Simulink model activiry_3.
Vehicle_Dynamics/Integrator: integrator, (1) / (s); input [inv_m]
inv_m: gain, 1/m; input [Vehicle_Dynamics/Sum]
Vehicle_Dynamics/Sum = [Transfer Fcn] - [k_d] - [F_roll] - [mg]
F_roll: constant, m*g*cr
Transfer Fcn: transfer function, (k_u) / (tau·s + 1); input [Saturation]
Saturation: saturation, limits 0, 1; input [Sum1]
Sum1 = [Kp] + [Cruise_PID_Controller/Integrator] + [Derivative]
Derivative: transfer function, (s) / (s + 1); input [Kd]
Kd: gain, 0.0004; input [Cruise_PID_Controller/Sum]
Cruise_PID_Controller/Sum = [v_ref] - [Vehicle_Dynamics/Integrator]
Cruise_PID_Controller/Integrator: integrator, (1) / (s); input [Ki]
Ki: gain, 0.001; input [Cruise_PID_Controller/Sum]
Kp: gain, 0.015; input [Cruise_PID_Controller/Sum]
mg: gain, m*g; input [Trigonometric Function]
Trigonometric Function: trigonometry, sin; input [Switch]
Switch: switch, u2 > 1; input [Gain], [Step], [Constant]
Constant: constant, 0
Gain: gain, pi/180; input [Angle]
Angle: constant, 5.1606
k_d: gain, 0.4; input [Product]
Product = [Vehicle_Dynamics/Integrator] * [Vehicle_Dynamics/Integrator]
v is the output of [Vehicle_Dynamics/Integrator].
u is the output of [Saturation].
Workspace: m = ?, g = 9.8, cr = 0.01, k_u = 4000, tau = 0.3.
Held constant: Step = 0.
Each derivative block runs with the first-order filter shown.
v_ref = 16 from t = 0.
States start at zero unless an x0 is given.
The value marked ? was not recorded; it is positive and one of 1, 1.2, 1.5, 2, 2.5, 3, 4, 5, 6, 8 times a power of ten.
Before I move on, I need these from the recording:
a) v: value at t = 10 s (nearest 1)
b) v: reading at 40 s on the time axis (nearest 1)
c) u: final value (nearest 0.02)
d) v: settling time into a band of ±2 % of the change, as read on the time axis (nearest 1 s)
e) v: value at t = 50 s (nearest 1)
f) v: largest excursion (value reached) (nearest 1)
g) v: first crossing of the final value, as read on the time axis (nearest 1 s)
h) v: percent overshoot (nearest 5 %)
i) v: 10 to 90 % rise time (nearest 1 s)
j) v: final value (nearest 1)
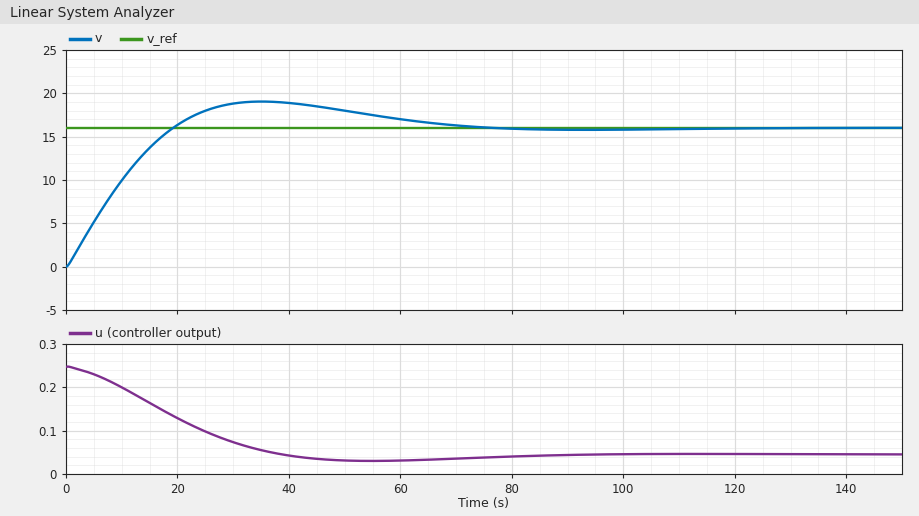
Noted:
10
19
0.04
70 s
18
19
19 s
20 %
14 s
16
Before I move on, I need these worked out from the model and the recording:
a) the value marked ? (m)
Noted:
800
